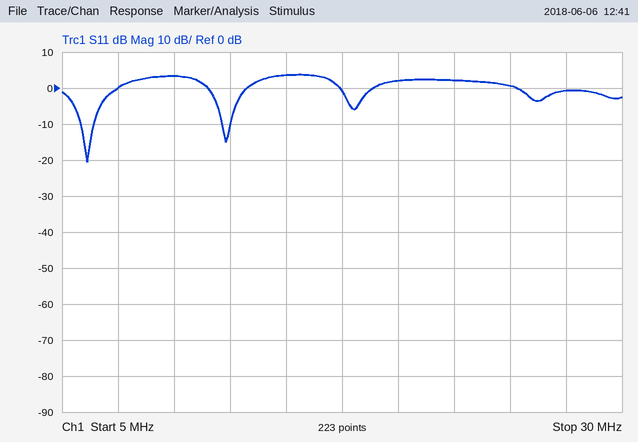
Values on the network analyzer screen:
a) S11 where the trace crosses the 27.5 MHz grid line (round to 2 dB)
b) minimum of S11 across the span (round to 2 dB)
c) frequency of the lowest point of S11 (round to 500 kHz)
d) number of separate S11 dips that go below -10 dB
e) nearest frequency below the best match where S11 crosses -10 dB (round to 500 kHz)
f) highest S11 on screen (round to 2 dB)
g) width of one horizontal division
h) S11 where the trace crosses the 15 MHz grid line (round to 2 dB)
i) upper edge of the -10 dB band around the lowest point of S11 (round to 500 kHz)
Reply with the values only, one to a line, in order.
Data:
0 dB
-20 dB
6.0 MHz
2
6.0 MHz
4 dB
2.5 MHz
4 dB
6.5 MHz
